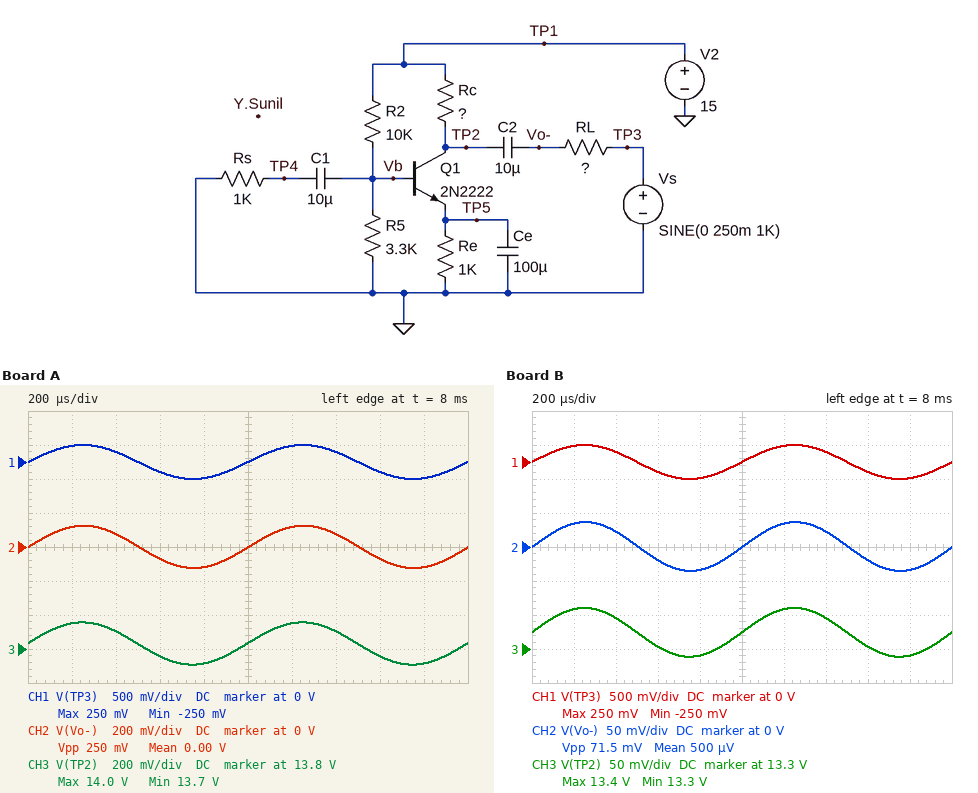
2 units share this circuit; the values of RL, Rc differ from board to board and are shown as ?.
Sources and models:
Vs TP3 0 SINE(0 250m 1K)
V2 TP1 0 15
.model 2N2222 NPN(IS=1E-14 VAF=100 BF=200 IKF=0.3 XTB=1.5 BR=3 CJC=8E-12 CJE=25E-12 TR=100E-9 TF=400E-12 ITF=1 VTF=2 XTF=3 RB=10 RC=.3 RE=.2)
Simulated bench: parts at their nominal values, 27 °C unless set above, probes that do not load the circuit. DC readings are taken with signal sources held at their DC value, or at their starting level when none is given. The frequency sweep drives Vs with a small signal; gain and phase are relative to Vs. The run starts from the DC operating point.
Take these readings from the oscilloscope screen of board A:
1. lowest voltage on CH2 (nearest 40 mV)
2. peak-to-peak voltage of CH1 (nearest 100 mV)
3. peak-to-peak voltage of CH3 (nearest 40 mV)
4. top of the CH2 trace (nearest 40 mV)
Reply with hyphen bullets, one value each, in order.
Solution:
- -120 mV
- 500 mV
- 240 mV
- 120 mV
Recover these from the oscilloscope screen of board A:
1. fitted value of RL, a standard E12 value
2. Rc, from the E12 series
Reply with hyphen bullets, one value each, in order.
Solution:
- 390 Ω
- 390 Ω
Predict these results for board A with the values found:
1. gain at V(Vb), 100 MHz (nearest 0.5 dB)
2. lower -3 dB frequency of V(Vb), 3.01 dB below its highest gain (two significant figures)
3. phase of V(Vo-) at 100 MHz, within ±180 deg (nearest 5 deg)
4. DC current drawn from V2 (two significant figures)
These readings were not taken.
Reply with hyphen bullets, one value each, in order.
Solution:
- -40.0 dB
- 1.9 MHz
- -15 deg
- 4.1 mA
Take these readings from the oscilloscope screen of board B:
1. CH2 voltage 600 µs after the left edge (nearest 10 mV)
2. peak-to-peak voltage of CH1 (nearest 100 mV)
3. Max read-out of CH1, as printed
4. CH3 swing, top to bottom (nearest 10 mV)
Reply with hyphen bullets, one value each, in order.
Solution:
- -20 mV
- 500 mV
- 250 mV
- 70 mV
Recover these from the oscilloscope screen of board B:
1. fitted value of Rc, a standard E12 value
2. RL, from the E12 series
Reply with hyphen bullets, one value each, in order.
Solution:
- 560 Ω
- 3.3 kΩ
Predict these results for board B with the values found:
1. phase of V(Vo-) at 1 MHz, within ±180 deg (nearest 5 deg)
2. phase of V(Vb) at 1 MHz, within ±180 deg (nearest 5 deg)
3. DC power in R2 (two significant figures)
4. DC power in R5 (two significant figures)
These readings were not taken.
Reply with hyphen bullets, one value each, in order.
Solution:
- -25 deg
- 50 deg
- 13 mW
- 4.1 mW
